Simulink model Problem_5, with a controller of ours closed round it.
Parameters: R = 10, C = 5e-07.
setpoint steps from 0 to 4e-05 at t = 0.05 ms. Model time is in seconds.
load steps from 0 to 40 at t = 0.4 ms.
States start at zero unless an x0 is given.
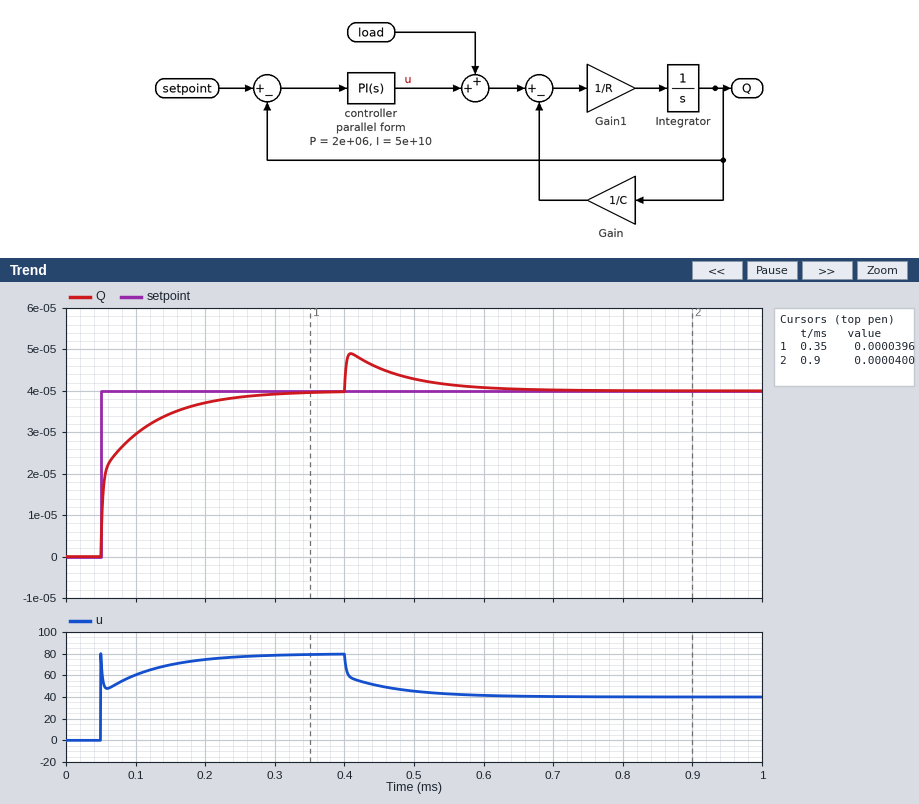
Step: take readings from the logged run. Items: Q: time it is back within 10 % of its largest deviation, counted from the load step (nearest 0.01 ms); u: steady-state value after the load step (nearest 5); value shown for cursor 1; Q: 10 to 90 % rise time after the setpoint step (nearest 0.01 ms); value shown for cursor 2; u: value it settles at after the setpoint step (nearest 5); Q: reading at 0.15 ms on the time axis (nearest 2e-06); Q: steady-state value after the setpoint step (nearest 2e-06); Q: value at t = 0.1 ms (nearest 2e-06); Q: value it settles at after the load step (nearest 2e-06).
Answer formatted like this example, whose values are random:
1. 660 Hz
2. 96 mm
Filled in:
1. 0.19 ms
2. 40
3. 0.0000396
4. 0.12 ms
5. 0.0000400
6. 80
7. 0.000034
8. 0.000040
9. 0.000030
10. 0.000040
